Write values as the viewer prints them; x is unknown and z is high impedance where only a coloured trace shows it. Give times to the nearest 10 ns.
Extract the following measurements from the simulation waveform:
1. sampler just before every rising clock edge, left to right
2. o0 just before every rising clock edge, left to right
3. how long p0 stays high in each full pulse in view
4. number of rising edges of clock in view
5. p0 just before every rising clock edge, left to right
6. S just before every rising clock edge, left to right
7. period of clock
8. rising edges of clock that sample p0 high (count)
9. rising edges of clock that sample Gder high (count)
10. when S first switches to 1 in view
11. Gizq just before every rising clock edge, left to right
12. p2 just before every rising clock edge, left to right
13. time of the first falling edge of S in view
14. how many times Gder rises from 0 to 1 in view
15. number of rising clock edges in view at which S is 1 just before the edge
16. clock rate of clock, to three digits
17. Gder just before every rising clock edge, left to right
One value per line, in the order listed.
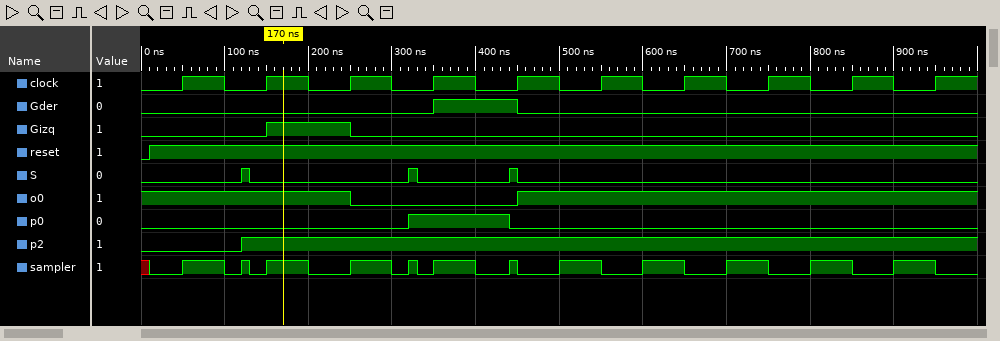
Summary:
0 0 0 0 1 1 1 1 1 1
1 1 1 0 0 1 1 1 1 1
120 ns
10
0 0 0 1 0 0 0 0 0 0
0 0 0 0 1 0 0 0 0 0
100 ns
1
1
120 ns
0 0 1 0 0 0 0 0 0 0
0 1 1 1 1 1 1 1 1 1
130 ns
1
1
10.0 MHz
0 0 0 0 1 0 0 0 0 0
